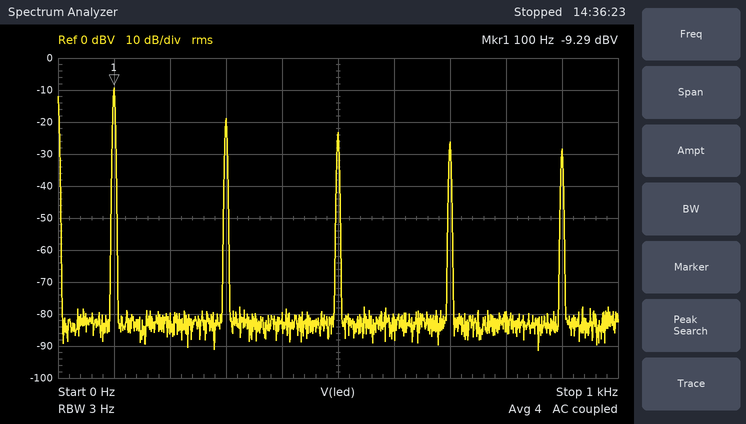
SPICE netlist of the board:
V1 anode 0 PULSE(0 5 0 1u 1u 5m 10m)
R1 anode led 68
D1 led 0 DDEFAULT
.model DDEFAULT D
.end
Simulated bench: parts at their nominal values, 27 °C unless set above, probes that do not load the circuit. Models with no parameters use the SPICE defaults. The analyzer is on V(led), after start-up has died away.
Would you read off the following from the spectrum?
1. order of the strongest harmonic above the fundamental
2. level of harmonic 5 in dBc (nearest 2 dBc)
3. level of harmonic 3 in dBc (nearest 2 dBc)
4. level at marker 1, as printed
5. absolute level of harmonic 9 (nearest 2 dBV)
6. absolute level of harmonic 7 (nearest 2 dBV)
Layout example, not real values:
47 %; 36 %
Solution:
3; -14 dBc; -10 dBc; -9.29 dBV; -28 dBV; -26 dBV
